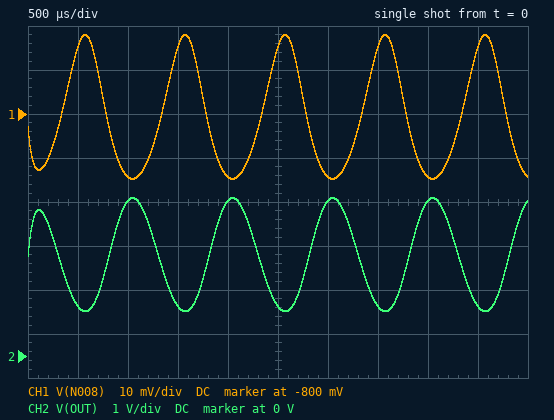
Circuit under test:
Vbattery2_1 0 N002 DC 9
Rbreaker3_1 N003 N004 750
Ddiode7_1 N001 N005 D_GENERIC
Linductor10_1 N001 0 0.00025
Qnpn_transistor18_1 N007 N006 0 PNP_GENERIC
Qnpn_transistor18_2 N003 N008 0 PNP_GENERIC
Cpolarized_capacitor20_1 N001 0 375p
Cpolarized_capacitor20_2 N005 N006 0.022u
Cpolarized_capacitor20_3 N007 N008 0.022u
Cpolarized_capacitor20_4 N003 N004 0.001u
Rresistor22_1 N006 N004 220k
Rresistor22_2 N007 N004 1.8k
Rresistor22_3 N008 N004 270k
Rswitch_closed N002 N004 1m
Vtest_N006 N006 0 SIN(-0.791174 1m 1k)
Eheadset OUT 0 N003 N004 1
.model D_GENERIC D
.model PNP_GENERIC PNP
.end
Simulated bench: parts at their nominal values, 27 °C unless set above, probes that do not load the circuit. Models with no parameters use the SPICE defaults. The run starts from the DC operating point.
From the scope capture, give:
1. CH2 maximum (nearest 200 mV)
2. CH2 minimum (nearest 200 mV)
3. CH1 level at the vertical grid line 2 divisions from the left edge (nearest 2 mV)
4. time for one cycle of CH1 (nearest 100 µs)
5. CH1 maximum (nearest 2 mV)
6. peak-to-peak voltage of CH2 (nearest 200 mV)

3.6 V
1.0 V
-814 mV
1.0 ms
-782 mV
2.6 V
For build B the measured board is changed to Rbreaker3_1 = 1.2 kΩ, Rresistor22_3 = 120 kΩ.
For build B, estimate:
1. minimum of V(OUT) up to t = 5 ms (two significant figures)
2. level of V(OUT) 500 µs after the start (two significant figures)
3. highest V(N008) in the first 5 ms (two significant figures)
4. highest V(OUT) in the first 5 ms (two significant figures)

6.1 V
6.2 V
-820 mV
8.8 V
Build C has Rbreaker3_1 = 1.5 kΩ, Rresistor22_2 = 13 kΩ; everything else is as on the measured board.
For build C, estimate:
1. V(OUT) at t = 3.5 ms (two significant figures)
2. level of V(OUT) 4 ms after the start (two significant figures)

4.5 V
4.6 V
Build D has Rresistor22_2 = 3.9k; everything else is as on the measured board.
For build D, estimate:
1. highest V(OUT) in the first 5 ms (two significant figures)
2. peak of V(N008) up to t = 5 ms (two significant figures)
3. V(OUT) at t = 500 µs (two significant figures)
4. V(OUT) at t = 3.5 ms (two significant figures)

4.8 V
-730 mV
430 mV
440 mV
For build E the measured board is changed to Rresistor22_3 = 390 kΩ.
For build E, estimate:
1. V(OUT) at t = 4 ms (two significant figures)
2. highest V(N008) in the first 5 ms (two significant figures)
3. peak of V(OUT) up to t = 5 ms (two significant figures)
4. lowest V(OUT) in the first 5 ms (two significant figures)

2.8 V
-760 mV
2.9 V
400 mV
